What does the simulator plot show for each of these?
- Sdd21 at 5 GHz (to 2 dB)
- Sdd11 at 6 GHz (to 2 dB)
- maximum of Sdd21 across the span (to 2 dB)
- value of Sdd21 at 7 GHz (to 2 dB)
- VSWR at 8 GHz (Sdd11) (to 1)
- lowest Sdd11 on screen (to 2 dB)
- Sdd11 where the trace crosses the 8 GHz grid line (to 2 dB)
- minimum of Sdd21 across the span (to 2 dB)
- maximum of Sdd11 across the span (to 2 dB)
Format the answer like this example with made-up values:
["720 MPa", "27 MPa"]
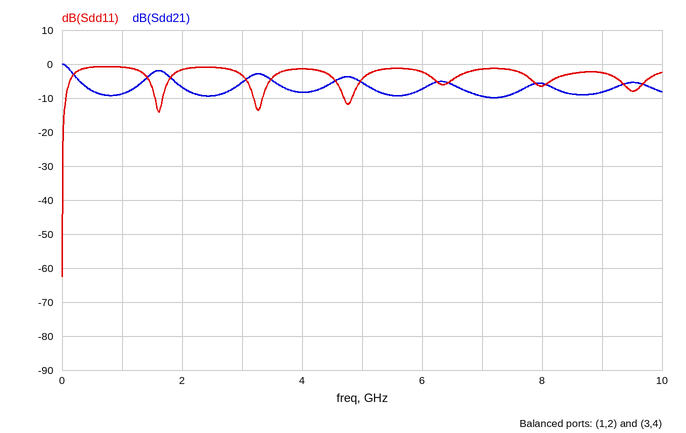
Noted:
["-6 dB", "-2 dB", "0 dB", "-10 dB", "3", "-62 dB", "-6 dB", "-10 dB", "0 dB"]
